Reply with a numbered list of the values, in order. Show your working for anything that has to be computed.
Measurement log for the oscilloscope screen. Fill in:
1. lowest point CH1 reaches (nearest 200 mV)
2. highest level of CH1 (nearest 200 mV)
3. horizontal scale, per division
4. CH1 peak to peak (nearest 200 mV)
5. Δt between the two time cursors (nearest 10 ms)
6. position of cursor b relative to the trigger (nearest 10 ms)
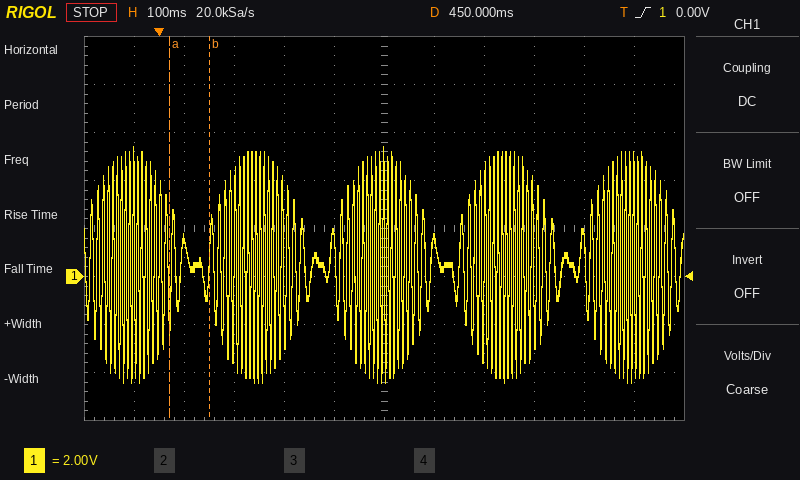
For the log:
1. -4.4 V
2. 5.4 V
3. 100 ms
4. 5.4 V − (-4.4 V) = 9.8 V
5. 80 ms
6. +100 ms
